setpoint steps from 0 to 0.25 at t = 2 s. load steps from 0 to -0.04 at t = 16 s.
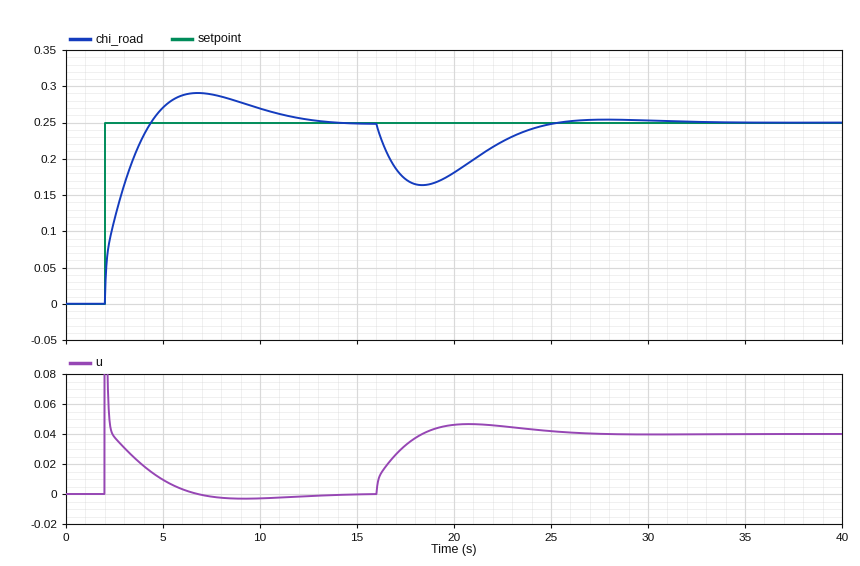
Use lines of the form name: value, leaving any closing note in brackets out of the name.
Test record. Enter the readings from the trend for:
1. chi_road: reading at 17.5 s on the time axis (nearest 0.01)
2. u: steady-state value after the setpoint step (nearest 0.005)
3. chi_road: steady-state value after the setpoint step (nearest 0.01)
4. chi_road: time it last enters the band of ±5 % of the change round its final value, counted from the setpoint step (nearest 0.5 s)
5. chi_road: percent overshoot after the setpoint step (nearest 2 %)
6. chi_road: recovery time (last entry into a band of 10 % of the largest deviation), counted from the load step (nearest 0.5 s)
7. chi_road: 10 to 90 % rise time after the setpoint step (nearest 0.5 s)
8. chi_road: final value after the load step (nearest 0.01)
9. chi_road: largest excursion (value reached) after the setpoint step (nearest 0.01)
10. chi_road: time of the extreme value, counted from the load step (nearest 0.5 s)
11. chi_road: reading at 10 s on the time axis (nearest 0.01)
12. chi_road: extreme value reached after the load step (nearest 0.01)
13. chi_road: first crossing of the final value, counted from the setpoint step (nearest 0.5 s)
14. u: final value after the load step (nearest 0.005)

chi_road: reading at 17.5 s on the time axis: 0.17
u: steady-state value after the setpoint step: 0.000
chi_road: steady-state value after the setpoint step: 0.25
chi_road: time it last enters the band of ±5 % of the change round its final value, counted from the setpoint step: 9.0 s
chi_road: percent overshoot after the setpoint step: 16 %
chi_road: recovery time (last entry into a band of 10 % of the largest deviation), counted from the load step: 8.0 s
chi_road: 10 to 90 % rise time after the setpoint step: 2.0 s
chi_road: final value after the load step: 0.25
chi_road: largest excursion (value reached) after the setpoint step: 0.29
chi_road: time of the extreme value, counted from the load step: 2.5 s
chi_road: reading at 10 s on the time axis: 0.27
chi_road: extreme value reached after the load step: 0.16
chi_road: first crossing of the final value, counted from the setpoint step: 2.5 s
u: final value after the load step: 0.040
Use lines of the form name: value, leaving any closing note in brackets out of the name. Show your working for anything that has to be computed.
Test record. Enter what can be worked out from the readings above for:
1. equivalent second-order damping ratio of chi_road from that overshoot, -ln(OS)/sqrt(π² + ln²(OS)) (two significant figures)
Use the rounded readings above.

equivalent second-order damping ratio of chi_road from that overshoot, -ln(OS)/sqrt(π² + ln²(OS)): ln(0.16) = -1.833; 1.833 / sqrt(9.870 + 3.358) = 0.50
